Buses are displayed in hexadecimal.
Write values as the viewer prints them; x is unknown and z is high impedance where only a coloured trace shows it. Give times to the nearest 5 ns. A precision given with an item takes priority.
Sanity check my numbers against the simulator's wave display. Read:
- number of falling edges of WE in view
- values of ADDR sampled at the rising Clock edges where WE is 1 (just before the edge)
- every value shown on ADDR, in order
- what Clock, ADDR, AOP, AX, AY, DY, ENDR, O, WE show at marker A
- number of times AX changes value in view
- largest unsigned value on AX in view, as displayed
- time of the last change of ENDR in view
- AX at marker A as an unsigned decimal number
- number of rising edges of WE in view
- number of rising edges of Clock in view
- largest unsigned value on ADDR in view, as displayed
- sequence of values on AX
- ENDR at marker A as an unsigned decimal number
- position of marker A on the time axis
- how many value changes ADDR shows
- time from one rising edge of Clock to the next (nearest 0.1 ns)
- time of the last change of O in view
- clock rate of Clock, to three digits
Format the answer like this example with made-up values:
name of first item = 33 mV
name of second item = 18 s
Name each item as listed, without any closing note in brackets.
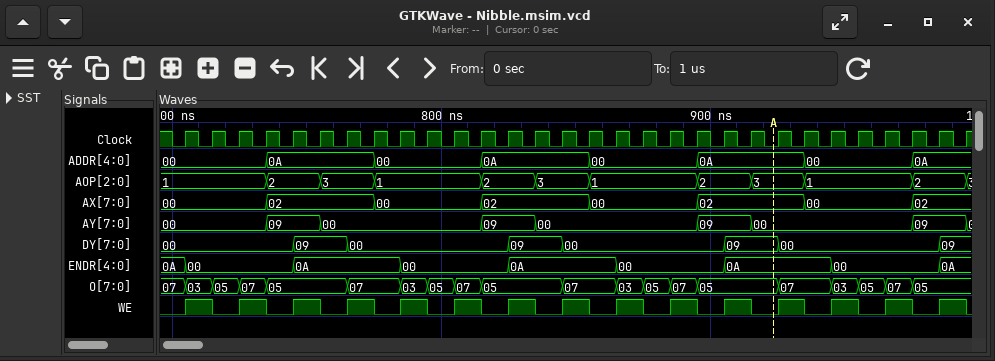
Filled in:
number of falling edges of WE in view = 15
values of ADDR sampled at the rising Clock edges where WE is 1 = 00, 00, 0A, 0A, 00, 00, 0A, 0A, 00, 00, 0A, 0A, 00, 00, 0A
every value shown on ADDR, in order = 00, 0A, 00, 0A, 00, 0A, 00, 0A
what Clock, ADDR, AOP, AX, AY, DY, ENDR, O, WE show at marker A = Clock=0, ADDR=0A, AOP=3, AX=02, AY=00, DY=09, ENDR=0A, O=05, WE=0
number of times AX changes value in view = 7
largest unsigned value on AX in view, as displayed = 02
time of the last change of ENDR in view = 985 ns
AX at marker A as an unsigned decimal number = 2
number of rising edges of WE in view = 15
number of rising edges of Clock in view = 30
largest unsigned value on ADDR in view, as displayed = 0A
sequence of values on AX = 00, 02, 00, 02, 00, 02, 00, 02
ENDR at marker A as an unsigned decimal number = 10
position of marker A on the time axis = 925 ns
how many value changes ADDR shows = 7
time from one rising edge of Clock to the next = 10 ns
time of the last change of O in view = 975 ns
clock rate of Clock, to three digits = 100 MHz
